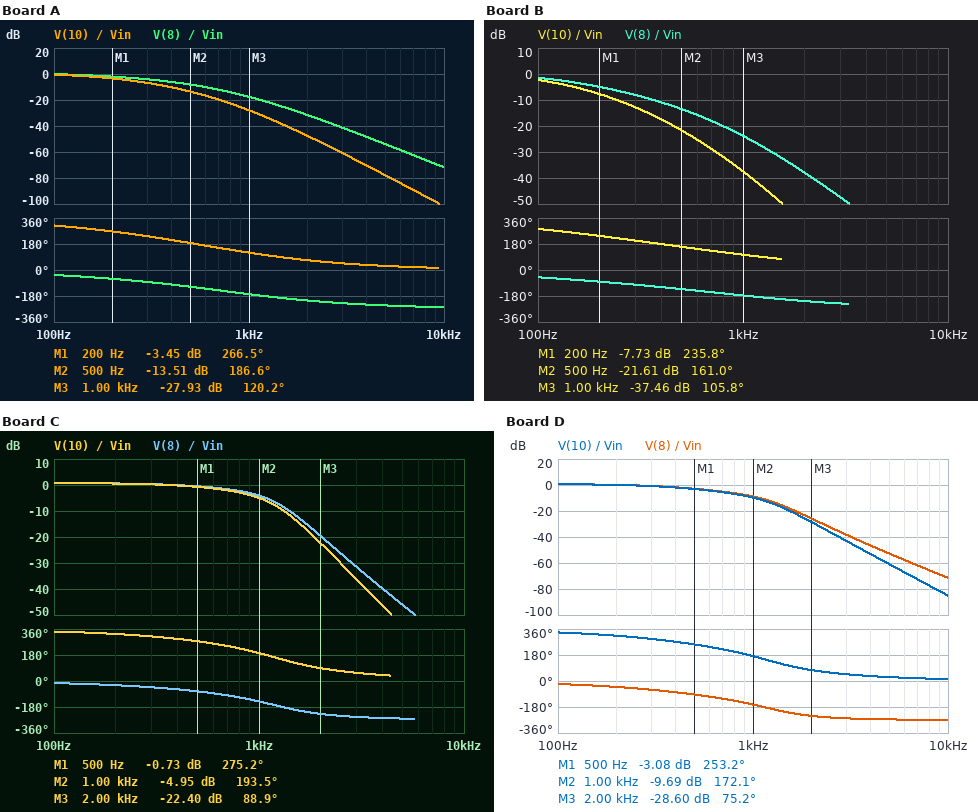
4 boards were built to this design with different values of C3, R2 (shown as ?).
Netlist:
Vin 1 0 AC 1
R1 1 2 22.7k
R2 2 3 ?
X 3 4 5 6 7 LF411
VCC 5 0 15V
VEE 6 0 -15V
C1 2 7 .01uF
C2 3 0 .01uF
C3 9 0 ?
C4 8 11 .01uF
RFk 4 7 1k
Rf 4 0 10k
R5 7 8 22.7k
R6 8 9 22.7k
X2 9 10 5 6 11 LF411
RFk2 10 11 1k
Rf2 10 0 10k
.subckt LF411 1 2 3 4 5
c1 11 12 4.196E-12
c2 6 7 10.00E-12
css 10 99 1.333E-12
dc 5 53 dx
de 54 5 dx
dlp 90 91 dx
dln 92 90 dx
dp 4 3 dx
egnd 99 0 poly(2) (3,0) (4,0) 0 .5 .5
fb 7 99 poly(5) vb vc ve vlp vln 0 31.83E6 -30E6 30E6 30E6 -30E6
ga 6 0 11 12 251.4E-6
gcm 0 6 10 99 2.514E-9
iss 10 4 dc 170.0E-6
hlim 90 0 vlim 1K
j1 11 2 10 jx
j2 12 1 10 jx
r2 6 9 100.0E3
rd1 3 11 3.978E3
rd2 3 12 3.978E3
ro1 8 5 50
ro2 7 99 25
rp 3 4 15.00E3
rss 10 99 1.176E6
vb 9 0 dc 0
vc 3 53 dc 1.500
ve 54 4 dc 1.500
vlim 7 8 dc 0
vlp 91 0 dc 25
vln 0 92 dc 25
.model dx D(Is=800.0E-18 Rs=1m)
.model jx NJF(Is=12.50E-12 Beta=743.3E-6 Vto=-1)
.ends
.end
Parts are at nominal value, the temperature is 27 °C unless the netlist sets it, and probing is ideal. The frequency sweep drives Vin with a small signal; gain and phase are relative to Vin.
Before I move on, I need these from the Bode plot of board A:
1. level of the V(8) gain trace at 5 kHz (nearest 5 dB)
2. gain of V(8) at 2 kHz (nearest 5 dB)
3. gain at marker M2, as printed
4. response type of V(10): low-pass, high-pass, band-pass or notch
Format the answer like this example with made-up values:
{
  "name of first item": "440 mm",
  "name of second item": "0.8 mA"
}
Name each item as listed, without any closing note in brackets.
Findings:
{
  "level of the V(8) gain trace at 5 kHz": "-55 dB",
  "gain of V(8) at 2 kHz": "-30 dB",
  "gain at marker M2, as printed": "-13.51 dB",
  "response type of V(10): low-pass, high-pass, band-pass or notch": "low-pass"
}
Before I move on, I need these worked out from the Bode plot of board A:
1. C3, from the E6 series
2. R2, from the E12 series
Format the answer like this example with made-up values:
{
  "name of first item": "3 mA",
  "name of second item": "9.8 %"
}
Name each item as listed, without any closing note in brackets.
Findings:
{
  "C3, from the E6 series": "22 nF",
  "R2, from the E12 series": "33 kΩ"
}
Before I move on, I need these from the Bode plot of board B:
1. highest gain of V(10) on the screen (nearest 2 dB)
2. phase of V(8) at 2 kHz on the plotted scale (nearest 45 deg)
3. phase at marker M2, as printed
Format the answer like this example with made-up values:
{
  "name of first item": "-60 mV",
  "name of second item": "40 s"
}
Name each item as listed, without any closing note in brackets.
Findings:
{
  "highest gain of V(10) on the screen": "-2 dB",
  "phase of V(8) at 2 kHz on the plotted scale": "-225 deg",
  "phase at marker M2, as printed": "161.0 deg"
}
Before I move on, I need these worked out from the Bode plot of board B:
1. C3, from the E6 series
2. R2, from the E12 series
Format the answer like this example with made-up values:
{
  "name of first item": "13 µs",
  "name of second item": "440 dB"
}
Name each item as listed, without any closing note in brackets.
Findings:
{
  "C3, from the E6 series": "33 nF",
  "R2, from the E12 series": "68 kΩ"
}
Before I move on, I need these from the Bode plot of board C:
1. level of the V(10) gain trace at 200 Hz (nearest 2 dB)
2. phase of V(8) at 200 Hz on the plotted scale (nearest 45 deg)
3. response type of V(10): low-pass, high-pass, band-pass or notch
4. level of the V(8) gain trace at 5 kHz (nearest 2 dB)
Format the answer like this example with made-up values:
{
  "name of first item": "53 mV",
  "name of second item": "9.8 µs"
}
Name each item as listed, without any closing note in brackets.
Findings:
{
  "level of the V(10) gain trace at 200 Hz": "0 dB",
  "phase of V(8) at 200 Hz on the plotted scale": "-45 deg",
  "response type of V(10): low-pass, high-pass, band-pass or notch": "low-pass",
  "level of the V(8) gain trace at 5 kHz": "-46 dB"
}
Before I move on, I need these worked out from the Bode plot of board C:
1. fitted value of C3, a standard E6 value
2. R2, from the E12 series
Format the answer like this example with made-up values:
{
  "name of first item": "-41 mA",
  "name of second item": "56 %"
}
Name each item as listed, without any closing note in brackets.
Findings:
{
  "fitted value of C3, a standard E6 value": "3.3 nF",
  "R2, from the E12 series": "15 kΩ"
}
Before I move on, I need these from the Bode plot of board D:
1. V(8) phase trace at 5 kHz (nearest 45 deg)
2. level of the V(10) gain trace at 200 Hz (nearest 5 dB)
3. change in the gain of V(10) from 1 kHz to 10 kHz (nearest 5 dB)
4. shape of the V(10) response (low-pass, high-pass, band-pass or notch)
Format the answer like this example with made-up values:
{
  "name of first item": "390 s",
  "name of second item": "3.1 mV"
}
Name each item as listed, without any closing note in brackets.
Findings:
{
  "V(8) phase trace at 5 kHz": "-270 deg",
  "level of the V(10) gain trace at 200 Hz": "0 dB",
  "change in the gain of V(10) from 1 kHz to 10 kHz": "-75 dB",
  "shape of the V(10) response": "low-pass"
}
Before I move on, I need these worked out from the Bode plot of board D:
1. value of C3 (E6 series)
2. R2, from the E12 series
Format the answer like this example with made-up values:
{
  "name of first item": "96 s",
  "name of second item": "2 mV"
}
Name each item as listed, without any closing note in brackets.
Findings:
{
  "value of C3": "3.3 nF",
  "R2, from the E12 series": "33 kΩ"
}
